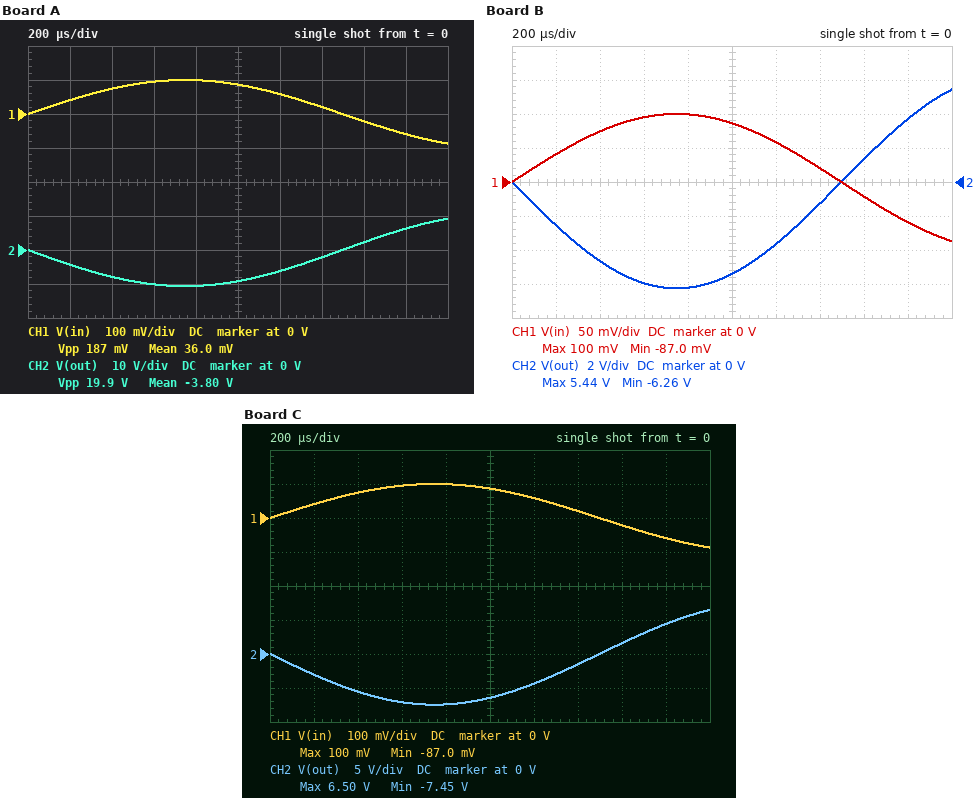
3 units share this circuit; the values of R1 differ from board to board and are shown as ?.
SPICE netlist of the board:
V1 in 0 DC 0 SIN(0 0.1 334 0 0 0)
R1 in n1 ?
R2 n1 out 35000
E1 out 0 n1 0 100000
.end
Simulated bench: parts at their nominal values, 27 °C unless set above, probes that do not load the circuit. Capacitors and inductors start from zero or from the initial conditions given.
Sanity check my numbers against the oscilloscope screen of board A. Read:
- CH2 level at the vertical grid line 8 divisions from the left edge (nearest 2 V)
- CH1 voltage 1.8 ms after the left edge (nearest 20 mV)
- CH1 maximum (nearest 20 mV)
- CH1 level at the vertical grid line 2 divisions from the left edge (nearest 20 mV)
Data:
2 V
-60 mV
100 mV
80 mV
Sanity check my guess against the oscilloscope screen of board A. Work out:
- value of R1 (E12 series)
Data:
330 Ω
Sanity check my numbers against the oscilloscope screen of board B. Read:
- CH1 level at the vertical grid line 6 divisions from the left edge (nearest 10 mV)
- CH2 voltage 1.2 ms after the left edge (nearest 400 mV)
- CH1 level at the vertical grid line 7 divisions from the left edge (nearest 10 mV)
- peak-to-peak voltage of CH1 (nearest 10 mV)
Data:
60 mV
-3.6 V
20 mV
190 mV
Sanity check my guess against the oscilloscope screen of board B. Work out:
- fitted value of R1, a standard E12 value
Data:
560 Ω
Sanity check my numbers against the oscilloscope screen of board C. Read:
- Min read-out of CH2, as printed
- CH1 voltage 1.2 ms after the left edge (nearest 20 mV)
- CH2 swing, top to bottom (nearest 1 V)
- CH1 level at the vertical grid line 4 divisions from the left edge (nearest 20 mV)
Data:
-7.45 V
60 mV
14 V
100 mV
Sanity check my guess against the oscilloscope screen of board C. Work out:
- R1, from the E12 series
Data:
470 Ω
